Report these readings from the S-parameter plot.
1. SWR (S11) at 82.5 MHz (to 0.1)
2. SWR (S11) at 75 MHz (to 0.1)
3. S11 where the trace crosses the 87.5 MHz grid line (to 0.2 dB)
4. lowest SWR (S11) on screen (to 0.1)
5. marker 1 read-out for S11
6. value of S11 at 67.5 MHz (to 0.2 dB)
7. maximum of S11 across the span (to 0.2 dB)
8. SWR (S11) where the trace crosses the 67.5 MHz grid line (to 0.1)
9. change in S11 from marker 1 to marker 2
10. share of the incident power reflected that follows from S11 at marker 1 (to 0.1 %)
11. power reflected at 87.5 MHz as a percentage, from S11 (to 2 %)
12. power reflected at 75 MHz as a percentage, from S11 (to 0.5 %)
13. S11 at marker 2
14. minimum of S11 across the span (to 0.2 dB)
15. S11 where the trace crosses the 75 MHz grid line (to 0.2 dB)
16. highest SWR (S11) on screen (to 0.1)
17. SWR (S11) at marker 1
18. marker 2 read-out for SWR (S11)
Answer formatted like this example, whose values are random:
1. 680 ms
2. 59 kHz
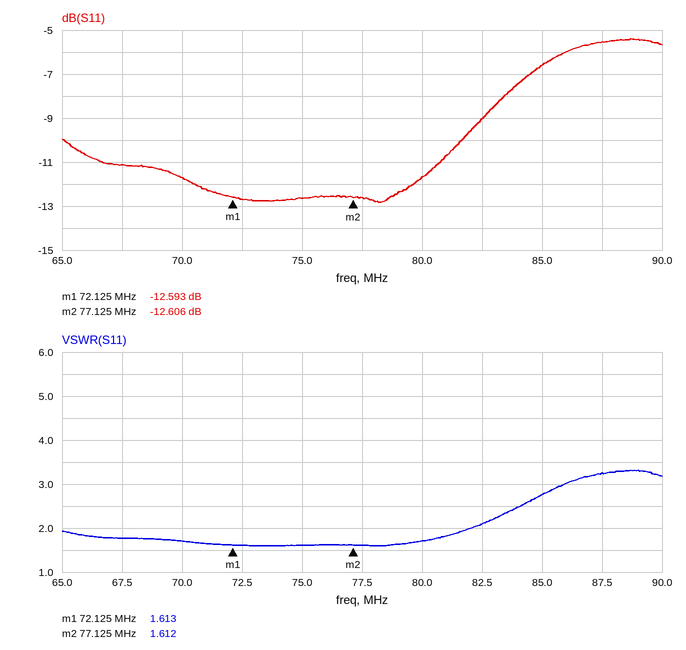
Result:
1. 2.1
2. 1.6
3. -5.6 dB
4. 1.6
5. -12.593 dB
6. -11.2 dB
7. -5.4 dB
8. 1.8
9. -0.013 dB
10. 5.5 %
11. 28 %
12. 5.5 %
13. -12.606 dB
14. -12.8 dB
15. -12.6 dB
16. 3.3
17. 1.613
18. 1.612
